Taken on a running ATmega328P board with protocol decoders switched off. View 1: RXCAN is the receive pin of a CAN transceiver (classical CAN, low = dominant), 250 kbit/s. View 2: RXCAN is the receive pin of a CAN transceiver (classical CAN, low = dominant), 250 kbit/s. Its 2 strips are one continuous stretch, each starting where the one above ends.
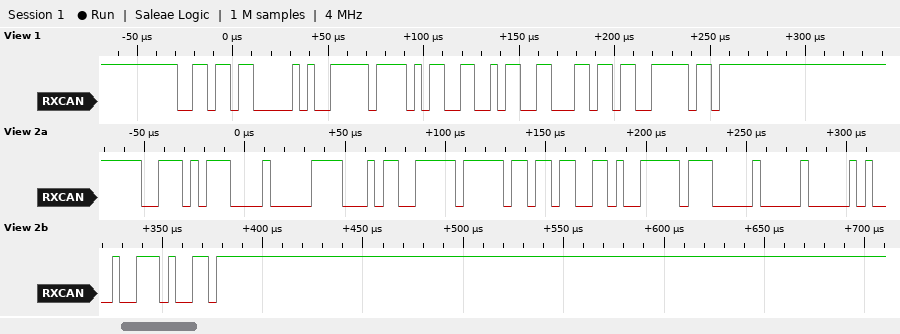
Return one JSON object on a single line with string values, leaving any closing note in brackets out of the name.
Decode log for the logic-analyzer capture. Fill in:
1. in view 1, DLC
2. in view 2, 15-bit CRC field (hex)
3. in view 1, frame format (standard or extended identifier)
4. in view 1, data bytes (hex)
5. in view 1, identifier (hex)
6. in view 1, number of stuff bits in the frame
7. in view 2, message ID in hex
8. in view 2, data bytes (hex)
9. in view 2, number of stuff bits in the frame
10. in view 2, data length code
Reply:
{"in view 1, DLC": "4", "in view 2, 15-bit CRC field": "0x44E9", "in view 1, frame format": "standard", "in view 1, data bytes": "FF AC CB 31", "in view 1, identifier": "0x36C", "in view 1, number of stuff bits in the frame": "3", "in view 2, message ID in hex": "0x3AE", "in view 2, data bytes": "38 B3 FF DB 34 FF 00 00", "in view 2, number of stuff bits in the frame": "7", "in view 2, data length code": "8"}
